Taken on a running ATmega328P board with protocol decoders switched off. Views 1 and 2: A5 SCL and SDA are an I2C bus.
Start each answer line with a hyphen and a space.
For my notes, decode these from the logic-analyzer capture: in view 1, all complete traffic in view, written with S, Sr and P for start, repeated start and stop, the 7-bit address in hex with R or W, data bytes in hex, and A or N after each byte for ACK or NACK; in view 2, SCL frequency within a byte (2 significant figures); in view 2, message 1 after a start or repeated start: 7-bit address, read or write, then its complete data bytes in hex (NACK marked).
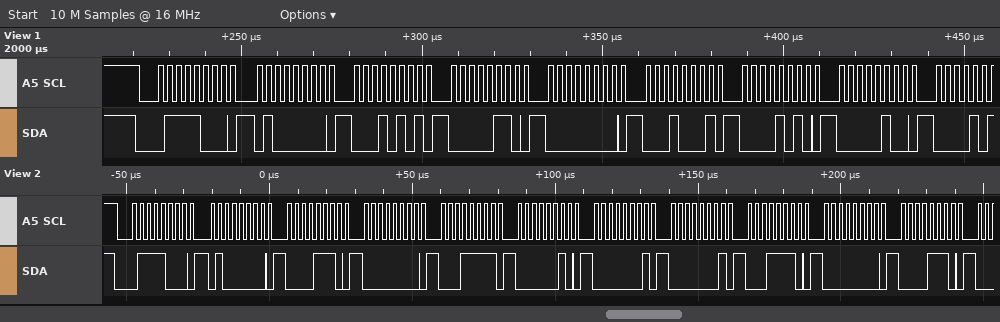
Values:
- S 3CW A 40 A 15 A 06 A 00 A 11 A 0A A 04 A
- 400 kHz
- 0x3C write: 40 0E 00 1F 02 01 01 1E 00 0E
